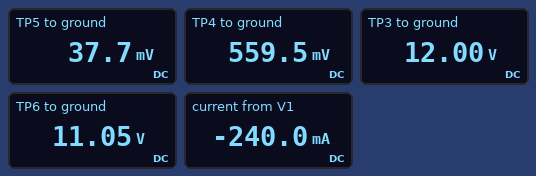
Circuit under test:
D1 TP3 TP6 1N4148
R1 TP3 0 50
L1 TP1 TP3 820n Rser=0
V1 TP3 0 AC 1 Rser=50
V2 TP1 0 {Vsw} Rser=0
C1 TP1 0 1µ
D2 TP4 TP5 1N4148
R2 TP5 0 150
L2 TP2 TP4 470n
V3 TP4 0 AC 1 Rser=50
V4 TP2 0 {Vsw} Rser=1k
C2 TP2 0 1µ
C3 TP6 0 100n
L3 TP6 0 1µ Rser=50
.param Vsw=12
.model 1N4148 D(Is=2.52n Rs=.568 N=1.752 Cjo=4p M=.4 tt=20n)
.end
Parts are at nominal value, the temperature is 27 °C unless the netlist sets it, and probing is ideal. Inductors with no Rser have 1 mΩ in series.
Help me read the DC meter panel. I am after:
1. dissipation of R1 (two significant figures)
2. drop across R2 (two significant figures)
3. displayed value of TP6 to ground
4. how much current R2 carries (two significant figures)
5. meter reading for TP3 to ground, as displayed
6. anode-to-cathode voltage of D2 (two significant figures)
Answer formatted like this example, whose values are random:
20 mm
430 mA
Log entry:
2.9 W
38 mV
11.05 V
250 µA
12.00 V
520 mV
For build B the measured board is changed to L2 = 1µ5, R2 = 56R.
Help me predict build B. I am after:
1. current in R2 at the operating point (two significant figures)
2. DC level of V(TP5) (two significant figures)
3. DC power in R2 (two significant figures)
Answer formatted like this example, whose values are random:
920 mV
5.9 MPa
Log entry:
340 µA
19 mV
6.6 µW
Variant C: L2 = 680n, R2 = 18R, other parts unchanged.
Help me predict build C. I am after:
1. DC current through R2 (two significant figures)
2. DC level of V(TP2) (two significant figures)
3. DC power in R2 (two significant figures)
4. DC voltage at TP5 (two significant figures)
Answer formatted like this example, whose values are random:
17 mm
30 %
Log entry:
410 µA
550 mV
3.1 µW
7.4 mV
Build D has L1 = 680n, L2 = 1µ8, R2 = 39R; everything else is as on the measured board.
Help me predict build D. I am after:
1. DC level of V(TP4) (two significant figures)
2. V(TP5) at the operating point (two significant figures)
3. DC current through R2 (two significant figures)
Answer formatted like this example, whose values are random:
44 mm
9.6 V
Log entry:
550 mV
14 mV
370 µA
